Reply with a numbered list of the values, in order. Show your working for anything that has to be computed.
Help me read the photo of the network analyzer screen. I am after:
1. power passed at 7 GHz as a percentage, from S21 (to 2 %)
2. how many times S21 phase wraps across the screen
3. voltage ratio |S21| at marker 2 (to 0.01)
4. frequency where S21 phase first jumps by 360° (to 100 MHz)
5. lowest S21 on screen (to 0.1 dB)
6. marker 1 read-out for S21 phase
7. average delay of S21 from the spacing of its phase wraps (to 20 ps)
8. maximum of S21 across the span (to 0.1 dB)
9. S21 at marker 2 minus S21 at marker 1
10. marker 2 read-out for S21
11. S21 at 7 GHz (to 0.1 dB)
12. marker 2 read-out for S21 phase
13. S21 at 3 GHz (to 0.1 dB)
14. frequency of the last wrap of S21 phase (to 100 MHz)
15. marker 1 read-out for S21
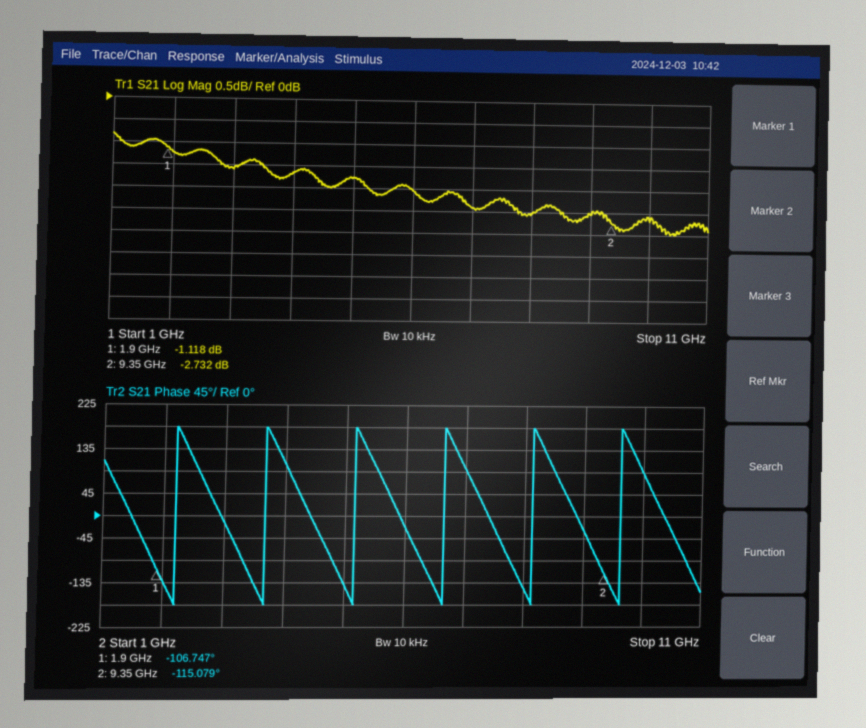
1. 10^(-2.4/10) ≈ 58 %
2. 6
3. 10^(-2.732/20) ≈ 0.73
4. 2.2 GHz
5. -3.0 dB
6. -106.747°
7. 5 cycles / (9.6 GHz − 2.2 GHz) ≈ 676 ps, so 680 ps to the nearest 20 ps
8. -0.8 dB
9. -2.732 − (-1.118) = -1.614 dB
10. -2.732 dB
11. -2.4 dB
12. -115.079°
13. -1.6 dB
14. 9.6 GHz
15. -1.118 dB
